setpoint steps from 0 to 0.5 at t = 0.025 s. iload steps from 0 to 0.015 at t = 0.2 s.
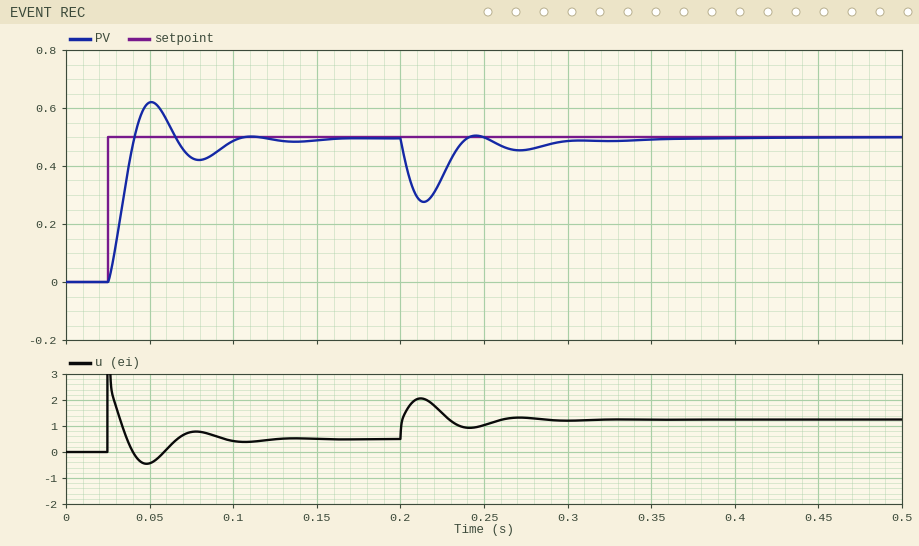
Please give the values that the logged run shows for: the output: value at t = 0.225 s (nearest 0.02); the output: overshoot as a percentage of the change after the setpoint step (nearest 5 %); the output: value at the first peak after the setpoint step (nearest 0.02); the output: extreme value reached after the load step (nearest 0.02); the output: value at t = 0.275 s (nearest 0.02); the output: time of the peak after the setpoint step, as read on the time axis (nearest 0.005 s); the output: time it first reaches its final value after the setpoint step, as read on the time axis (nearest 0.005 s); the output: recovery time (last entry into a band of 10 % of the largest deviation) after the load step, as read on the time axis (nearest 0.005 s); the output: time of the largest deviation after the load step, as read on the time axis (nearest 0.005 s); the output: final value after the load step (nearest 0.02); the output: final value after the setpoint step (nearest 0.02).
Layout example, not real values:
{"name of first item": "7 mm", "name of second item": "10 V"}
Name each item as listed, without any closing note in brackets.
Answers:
{"the output: value at t = 0.225 s": "0.36", "the output: overshoot as a percentage of the change after the setpoint step": "25 %", "the output: value at the first peak after the setpoint step": "0.62", "the output: extreme value reached after the load step": "0.28", "the output: value at t = 0.275 s": "0.46", "the output: time of the peak after the setpoint step, as read on the time axis": "0.050 s", "the output: time it first reaches its final value after the setpoint step, as read on the time axis": "0.040 s", "the output: recovery time (last entry into a band of 10 % of the largest deviation) after the load step, as read on the time axis": "0.290 s", "the output: time of the largest deviation after the load step, as read on the time axis": "0.215 s", "the output: final value after the load step": "0.50", "the output: final value after the setpoint step": "0.50"}
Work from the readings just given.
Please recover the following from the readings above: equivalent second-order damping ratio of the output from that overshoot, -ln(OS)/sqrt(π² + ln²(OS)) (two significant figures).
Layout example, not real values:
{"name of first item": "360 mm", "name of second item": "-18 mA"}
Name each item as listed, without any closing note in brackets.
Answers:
{"equivalent second-order damping ratio of the output from that overshoot, -ln(OS)/sqrt(π² + ln²(OS))": "0.40"}
